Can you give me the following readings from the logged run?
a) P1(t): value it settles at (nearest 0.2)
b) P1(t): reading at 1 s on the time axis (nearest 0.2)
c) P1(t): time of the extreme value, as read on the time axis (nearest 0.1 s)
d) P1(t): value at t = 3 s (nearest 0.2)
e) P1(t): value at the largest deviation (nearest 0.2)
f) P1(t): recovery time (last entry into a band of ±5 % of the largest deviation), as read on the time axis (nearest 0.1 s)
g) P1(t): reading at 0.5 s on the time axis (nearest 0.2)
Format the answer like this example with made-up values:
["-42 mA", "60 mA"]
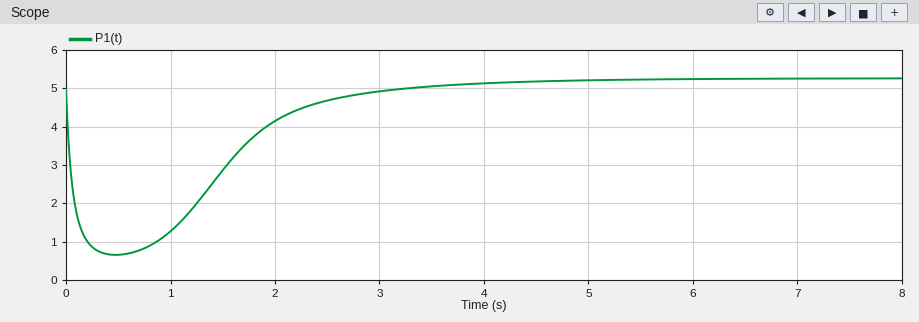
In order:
["5.2", "1.2", "0.5 s", "5.0", "0.6", "3.5 s", "0.6"]
